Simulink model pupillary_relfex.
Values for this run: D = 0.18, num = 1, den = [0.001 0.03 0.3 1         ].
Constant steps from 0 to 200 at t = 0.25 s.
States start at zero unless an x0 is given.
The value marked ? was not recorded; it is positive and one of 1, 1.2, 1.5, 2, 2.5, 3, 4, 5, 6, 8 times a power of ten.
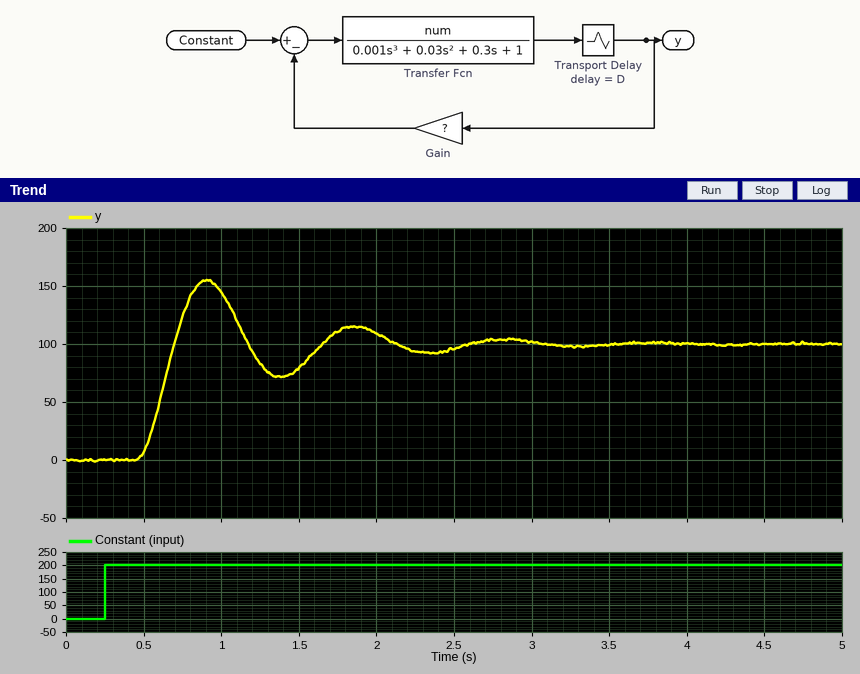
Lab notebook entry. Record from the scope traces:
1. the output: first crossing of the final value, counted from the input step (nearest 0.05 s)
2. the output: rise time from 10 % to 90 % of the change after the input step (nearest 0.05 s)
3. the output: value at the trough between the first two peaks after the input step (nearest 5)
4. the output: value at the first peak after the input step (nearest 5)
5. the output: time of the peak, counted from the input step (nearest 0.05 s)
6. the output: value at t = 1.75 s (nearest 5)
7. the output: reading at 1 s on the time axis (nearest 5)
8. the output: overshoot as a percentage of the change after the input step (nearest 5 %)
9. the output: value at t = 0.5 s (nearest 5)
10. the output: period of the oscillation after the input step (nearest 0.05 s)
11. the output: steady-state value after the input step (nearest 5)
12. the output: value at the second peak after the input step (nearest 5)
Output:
0.45 s
0.15 s
70
155
0.65 s
110
145
55 %
5
0.95 s
100
115
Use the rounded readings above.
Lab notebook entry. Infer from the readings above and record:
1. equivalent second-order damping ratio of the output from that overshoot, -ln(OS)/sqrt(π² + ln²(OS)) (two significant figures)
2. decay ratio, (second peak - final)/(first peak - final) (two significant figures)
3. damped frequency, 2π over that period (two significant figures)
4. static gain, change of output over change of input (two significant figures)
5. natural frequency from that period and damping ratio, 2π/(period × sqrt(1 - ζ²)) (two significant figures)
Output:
0.19
0.27
6.6 rad/s
0.50
6.7 rad/s
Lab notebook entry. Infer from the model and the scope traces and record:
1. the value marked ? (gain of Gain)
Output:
1
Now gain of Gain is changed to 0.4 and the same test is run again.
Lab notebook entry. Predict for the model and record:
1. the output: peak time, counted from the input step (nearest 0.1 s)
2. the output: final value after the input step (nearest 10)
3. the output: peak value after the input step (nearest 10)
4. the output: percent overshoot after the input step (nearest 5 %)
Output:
0.7 s
140
170
20 %
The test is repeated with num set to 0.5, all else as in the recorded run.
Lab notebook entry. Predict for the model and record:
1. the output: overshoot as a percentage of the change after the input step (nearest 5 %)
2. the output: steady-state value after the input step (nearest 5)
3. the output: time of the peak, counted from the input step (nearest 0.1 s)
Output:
25 %
65
0.7 s
